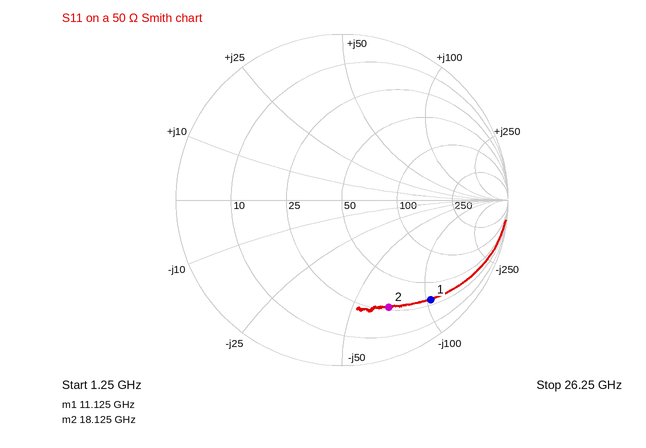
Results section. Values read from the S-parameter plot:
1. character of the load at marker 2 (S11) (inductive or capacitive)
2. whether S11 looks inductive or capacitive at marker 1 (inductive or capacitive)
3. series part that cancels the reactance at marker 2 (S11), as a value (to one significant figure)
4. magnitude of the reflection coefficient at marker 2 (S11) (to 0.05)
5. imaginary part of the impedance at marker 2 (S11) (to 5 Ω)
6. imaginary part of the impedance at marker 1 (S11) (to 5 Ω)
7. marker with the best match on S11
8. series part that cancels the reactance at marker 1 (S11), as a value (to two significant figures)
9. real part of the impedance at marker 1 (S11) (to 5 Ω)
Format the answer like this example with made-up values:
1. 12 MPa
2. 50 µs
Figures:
1. capacitive
2. capacitive
3. 600 pH
4. 0.70
5. -70 Ω
6. -105 Ω
7. marker 2
8. 1.5 nH
9. 30 Ω
